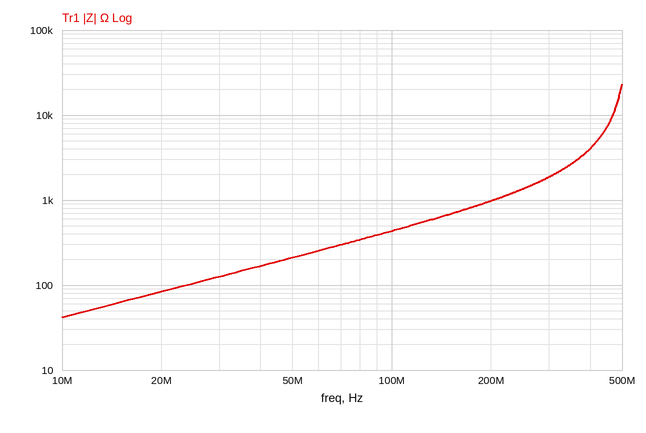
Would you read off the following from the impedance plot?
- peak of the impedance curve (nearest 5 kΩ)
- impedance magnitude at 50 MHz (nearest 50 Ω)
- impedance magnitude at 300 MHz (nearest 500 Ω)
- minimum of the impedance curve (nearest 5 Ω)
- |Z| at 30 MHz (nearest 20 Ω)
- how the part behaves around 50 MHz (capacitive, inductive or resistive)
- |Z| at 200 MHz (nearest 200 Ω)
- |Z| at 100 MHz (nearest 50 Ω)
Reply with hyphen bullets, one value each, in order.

- 25 kΩ
- 200 Ω
- 2.0 kΩ
- 40 Ω
- 120 Ω
- inductive
- 1.0 kΩ
- 450 Ω
